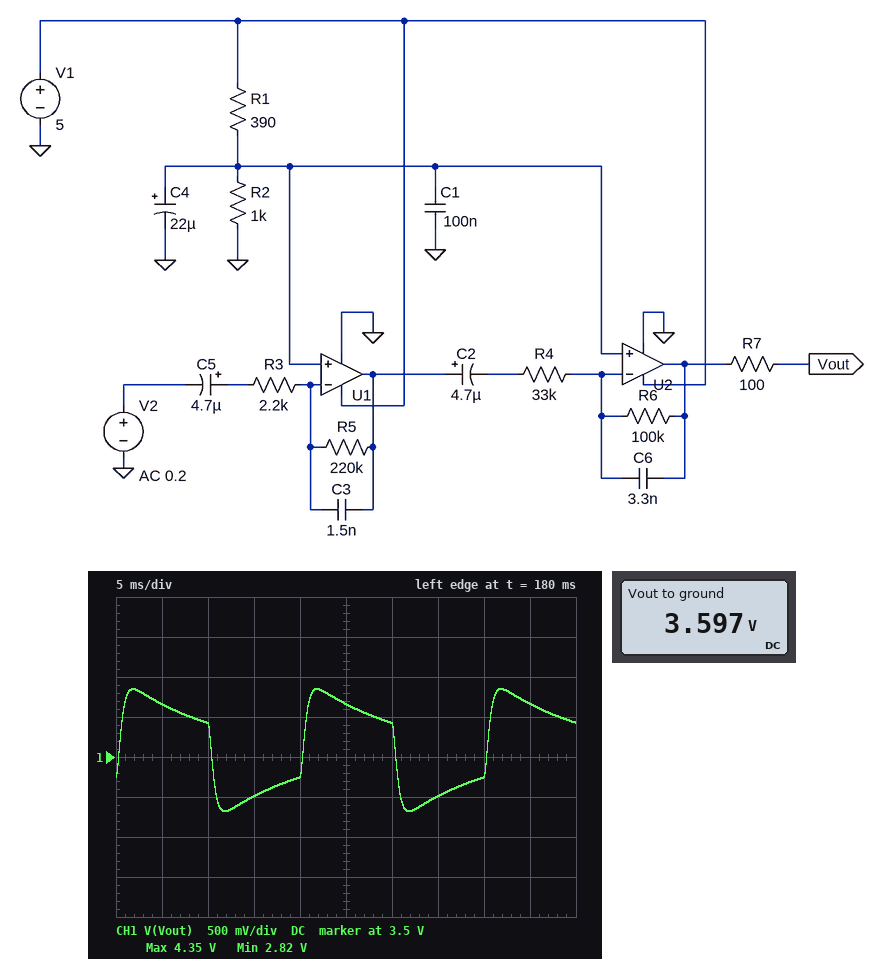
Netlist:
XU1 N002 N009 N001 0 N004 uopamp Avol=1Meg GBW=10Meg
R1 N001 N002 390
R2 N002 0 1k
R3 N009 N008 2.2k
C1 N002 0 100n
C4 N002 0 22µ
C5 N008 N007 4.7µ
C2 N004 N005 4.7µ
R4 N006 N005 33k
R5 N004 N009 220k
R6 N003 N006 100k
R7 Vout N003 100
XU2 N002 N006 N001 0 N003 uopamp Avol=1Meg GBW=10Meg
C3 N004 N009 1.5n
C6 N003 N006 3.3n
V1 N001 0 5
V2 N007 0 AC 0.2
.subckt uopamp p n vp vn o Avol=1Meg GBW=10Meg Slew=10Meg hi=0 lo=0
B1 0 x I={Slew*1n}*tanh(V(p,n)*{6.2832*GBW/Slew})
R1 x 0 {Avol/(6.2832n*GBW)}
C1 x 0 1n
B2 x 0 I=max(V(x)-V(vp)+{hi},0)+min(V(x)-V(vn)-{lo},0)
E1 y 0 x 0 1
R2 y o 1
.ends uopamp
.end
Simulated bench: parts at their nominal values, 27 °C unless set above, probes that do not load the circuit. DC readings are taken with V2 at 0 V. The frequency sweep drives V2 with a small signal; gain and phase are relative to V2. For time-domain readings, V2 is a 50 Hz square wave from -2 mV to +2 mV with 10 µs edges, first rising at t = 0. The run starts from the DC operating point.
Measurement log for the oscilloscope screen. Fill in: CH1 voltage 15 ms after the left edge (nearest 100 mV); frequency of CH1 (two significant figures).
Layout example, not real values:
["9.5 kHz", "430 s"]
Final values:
["3.0 V", "50 Hz"]
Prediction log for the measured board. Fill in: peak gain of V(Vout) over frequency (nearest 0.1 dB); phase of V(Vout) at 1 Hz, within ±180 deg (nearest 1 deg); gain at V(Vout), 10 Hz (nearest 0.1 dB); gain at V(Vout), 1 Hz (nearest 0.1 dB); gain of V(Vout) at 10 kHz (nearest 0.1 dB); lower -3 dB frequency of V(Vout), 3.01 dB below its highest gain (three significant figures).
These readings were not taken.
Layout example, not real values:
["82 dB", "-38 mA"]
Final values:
["49.2 dB", "132 deg", "44.3 dB", "22.7 dB", "-3.1 dB", "14.2 Hz"]
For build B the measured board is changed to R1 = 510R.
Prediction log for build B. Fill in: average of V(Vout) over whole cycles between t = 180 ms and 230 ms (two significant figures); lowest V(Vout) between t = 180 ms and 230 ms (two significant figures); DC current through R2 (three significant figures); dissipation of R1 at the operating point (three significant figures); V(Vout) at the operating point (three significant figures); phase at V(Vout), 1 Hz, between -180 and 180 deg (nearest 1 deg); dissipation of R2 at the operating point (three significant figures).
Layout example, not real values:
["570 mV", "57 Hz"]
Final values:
["3.3 V", "2.5 V", "3.31 mA", "5.59 mW", "3.31 V", "132 deg", "11.0 mW"]
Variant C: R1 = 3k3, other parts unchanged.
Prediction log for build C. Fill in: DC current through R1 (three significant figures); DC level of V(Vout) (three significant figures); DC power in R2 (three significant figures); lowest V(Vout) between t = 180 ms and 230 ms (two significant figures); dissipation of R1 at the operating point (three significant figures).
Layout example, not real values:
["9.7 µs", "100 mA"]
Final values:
["1.16 mA", "1.16 V", "1.35 mW", "390 mV", "4.46 mW"]
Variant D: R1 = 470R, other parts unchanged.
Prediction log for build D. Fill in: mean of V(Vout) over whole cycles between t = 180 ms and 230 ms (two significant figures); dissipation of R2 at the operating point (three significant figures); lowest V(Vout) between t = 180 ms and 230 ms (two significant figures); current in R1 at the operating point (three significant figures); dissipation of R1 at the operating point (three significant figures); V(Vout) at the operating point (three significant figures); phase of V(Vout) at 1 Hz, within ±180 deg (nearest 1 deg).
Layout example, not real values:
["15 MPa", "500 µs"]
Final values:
["3.4 V", "11.6 mW", "2.6 V", "3.40 mA", "5.44 mW", "3.40 V", "132 deg"]
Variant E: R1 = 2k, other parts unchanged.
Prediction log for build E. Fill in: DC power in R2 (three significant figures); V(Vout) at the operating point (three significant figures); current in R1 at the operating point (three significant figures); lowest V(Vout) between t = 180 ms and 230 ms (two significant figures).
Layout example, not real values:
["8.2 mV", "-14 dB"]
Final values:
["2.78 mW", "1.67 V", "1.67 mA", "890 mV"]
